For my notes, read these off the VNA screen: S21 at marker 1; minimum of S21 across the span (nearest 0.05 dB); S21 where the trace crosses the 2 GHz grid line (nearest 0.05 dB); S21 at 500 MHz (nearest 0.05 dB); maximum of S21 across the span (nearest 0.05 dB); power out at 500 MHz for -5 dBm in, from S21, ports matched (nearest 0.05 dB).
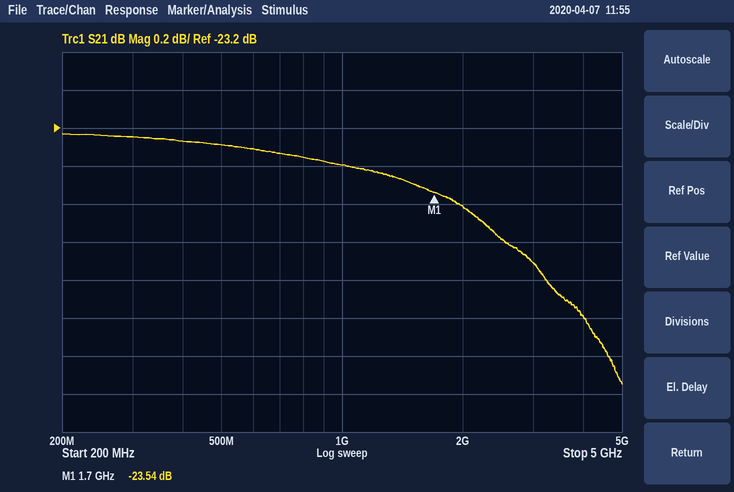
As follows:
-23.54 dB
-24.55 dB
-23.60 dB
-23.30 dB
-23.25 dB
-28.30 dBm
